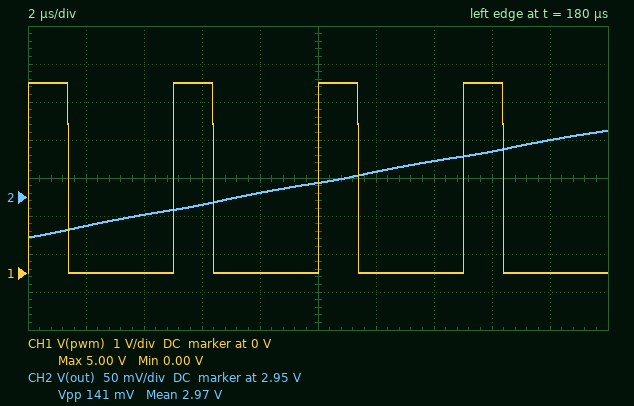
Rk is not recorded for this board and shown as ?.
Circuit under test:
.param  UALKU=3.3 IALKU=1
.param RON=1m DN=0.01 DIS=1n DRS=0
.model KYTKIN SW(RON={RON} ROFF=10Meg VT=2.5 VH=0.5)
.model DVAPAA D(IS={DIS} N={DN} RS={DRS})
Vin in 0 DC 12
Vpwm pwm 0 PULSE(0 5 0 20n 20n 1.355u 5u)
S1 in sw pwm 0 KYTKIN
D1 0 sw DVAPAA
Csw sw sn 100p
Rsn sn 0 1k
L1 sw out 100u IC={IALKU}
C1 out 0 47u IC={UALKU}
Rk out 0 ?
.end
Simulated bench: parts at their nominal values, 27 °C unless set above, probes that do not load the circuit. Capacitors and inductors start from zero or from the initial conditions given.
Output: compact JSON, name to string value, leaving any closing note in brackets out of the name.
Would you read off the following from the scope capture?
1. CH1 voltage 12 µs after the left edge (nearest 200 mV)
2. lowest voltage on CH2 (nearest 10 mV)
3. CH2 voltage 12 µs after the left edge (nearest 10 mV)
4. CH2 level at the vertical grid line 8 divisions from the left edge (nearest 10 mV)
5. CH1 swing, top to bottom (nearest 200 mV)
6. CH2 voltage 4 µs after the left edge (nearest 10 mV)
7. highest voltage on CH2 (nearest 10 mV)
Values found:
{"CH1 voltage 12 µs after the left edge": "0 V", "lowest voltage on CH2": "2.90 V", "CH2 voltage 12 µs after the left edge": "2.98 V", "CH2 level at the vertical grid line 8 divisions from the left edge": "3.01 V", "CH1 swing, top to bottom": "5.0 V", "CH2 voltage 4 µs after the left edge": "2.93 V", "highest voltage on CH2": "3.04 V"}
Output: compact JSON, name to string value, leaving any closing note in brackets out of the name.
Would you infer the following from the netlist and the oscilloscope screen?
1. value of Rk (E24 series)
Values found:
{"value of Rk": "1.5 Ω"}
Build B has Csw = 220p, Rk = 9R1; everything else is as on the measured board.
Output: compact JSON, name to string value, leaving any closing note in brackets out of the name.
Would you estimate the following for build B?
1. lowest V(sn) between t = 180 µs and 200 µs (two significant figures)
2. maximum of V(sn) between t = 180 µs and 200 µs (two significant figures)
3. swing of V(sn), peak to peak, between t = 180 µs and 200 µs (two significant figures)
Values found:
{"lowest V(sn) between t = 180 µs and 200 µs": "-12 V", "maximum of V(sn) between t = 180 µs and 200 µs": "8.4 V", "swing of V(sn), peak to peak, between t = 180 µs and 200 µs": "20 V"}
